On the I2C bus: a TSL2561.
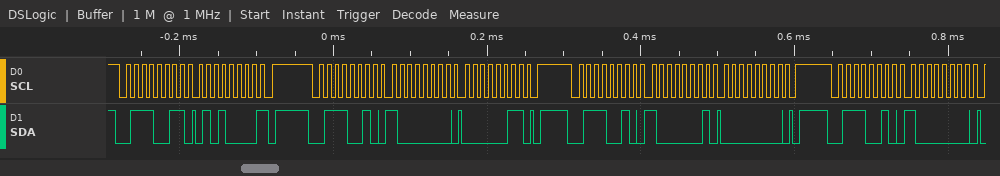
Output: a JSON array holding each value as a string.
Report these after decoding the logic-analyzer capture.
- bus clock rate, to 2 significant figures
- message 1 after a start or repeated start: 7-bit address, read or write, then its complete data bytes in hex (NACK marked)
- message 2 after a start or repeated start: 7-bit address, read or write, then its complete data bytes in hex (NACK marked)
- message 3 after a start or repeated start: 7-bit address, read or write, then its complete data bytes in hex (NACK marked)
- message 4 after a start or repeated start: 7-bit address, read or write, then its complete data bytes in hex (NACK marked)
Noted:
["100 kHz", "0x39 read: 50 NACK", "0x39 write: 80 03", "0x39 write: 81 00", "0x39 write: 80"]
